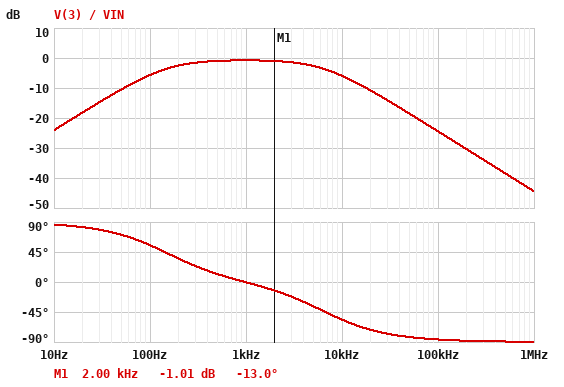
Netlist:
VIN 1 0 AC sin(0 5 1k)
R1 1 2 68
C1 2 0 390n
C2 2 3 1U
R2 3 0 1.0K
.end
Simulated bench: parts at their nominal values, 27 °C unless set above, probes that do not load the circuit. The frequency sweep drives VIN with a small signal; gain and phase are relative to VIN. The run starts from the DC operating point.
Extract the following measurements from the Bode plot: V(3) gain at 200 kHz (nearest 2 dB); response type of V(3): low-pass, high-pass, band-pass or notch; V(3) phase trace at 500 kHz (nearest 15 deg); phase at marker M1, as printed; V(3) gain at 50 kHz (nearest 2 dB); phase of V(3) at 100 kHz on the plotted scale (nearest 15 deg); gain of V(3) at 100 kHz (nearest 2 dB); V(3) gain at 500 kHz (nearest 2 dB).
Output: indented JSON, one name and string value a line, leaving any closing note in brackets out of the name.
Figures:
{
  "V(3) gain at 200 kHz": "-30 dB",
  "response type of V(3): low-pass, high-pass, band-pass or notch": "band-pass",
  "V(3) phase trace at 500 kHz": "-90 deg",
  "phase at marker M1, as printed": "-13.0 deg",
  "V(3) gain at 50 kHz": "-18 dB",
  "phase of V(3) at 100 kHz on the plotted scale": "-90 deg",
  "gain of V(3) at 100 kHz": "-24 dB",
  "V(3) gain at 500 kHz": "-38 dB"
}
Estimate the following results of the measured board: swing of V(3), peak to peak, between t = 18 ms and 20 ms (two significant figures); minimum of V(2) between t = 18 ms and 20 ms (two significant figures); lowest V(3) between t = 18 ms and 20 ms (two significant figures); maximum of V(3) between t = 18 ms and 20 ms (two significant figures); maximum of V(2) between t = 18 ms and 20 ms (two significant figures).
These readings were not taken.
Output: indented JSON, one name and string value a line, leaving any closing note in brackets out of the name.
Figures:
{
  "swing of V(3), peak to peak, between t = 18 ms and 20 ms": "9.1 V",
  "minimum of V(2) between t = 18 ms and 20 ms": "-4.6 V",
  "lowest V(3) between t = 18 ms and 20 ms": "-4.6 V",
  "maximum of V(3) between t = 18 ms and 20 ms": "4.6 V",
  "maximum of V(2) between t = 18 ms and 20 ms": "4.6 V"
}
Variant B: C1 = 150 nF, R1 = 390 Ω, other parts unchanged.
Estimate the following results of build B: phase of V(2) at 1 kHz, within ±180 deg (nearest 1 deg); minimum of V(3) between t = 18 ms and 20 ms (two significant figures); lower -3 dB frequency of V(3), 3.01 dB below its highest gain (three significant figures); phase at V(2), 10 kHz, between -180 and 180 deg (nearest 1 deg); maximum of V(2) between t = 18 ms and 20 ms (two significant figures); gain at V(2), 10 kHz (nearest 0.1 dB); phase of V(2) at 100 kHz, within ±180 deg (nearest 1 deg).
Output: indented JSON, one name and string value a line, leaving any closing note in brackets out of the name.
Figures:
{
  "phase of V(2) at 1 kHz, within ±180 deg": "-17 deg",
  "minimum of V(3) between t = 18 ms and 20 ms": "-3.4 V",
  "lower -3 dB frequency of V(3), 3.01 dB below its highest gain": "107 Hz",
  "phase at V(2), 10 kHz, between -180 and 180 deg": "-69 deg",
  "maximum of V(2) between t = 18 ms and 20 ms": "3.5 V",
  "gain at V(2), 10 kHz": "-11.9 dB",
  "phase of V(2) at 100 kHz, within ±180 deg": "-88 deg"
}
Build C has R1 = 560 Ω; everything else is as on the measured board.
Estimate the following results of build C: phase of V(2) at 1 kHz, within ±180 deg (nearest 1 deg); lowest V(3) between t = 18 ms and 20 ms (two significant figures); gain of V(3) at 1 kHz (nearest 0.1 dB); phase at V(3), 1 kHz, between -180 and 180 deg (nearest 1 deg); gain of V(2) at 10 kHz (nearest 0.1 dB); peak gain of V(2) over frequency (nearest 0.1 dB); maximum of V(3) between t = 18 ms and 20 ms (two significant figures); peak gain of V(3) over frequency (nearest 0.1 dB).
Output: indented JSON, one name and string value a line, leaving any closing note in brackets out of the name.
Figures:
{
  "phase of V(2) at 1 kHz, within ±180 deg": "-43 deg",
  "lowest V(3) between t = 18 ms and 20 ms": "-2.3 V",
  "gain of V(3) at 1 kHz": "-6.7 dB",
  "phase at V(3), 1 kHz, between -180 and 180 deg": "-34 deg",
  "gain of V(2) at 10 kHz": "-22.8 dB",
  "peak gain of V(2) over frequency": "0 dB",
  "maximum of V(3) between t = 18 ms and 20 ms": "2.3 V",
  "peak gain of V(3) over frequency": "-5.0 dB"
}
